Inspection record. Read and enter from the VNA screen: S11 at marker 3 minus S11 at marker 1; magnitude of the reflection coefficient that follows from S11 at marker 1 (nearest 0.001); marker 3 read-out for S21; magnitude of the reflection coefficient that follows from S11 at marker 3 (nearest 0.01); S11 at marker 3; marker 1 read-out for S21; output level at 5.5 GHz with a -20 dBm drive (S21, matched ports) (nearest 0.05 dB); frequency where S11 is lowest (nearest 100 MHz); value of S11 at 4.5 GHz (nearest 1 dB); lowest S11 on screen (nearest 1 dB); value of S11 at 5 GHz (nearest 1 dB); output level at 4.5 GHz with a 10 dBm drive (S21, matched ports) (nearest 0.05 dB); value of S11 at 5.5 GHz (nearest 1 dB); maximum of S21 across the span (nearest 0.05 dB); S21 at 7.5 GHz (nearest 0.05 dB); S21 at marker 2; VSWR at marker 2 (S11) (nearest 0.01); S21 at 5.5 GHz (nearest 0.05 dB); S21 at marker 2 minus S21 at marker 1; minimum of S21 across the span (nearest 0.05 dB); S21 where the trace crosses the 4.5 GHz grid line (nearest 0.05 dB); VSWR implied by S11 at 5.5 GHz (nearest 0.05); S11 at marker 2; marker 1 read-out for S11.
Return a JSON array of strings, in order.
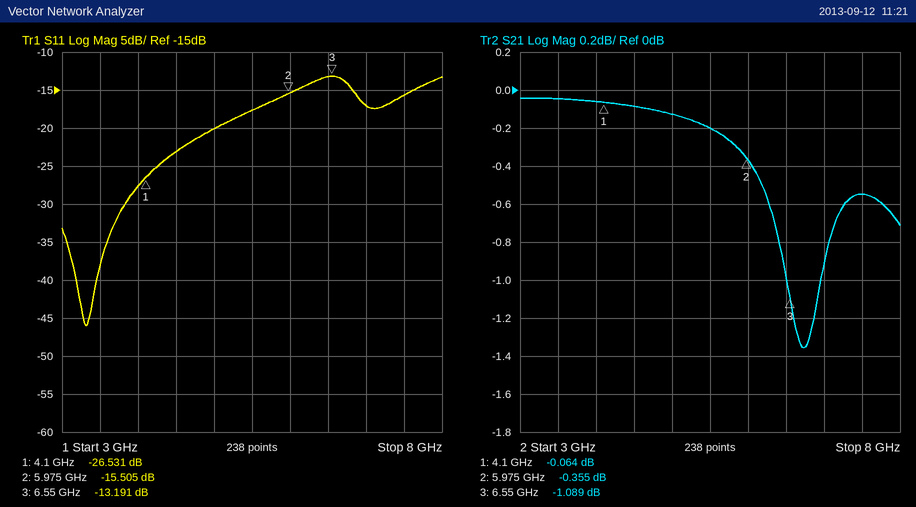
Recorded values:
["13.340 dB", "0.047", "-1.089 dB", "0.22", "-13.191 dB", "-0.064 dB", "-20.20 dBm", "3.3 GHz", "-23 dB", "-46 dB", "-20 dB", "9.90 dBm", "-18 dB", "-0.05 dB", "-0.55 dB", "-0.355 dB", "1.40", "-0.20 dB", "-0.291 dB", "-1.35 dB", "-0.10 dB", "1.30", "-15.505 dB", "-26.531 dB"]
